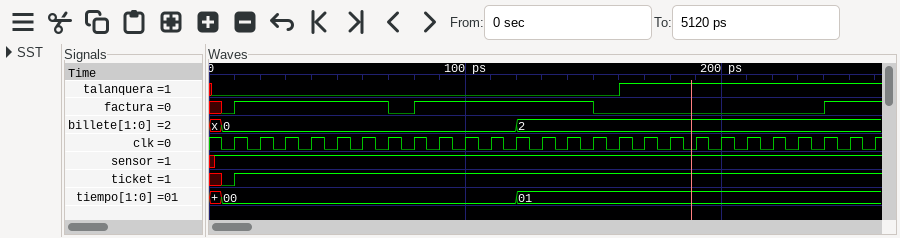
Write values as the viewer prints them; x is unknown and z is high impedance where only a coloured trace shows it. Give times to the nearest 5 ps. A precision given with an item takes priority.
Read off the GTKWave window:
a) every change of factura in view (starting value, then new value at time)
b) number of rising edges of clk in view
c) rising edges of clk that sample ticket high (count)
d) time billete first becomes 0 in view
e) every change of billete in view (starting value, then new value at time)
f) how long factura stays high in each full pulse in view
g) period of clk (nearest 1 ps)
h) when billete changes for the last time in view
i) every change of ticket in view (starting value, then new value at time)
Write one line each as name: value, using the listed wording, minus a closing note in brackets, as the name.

every change of factura in view: x, 0 at 5 ps, 1 at 10 ps, 0 at 70 ps, 1 at 80 ps, 0 at 150 ps, 1 at 240 ps
number of rising edges of clk in view: 26
rising edges of clk that sample ticket high: 25
time billete first becomes 0 in view: 5 ps
every change of billete in view: x, 0 at 5 ps, 2 at 120 ps
how long factura stays high in each full pulse in view: 60 ps, 70 ps
period of clk: 10 ps
when billete changes for the last time in view: 120 ps
every change of ticket in view: x, 0 at 5 ps, 1 at 10 ps
